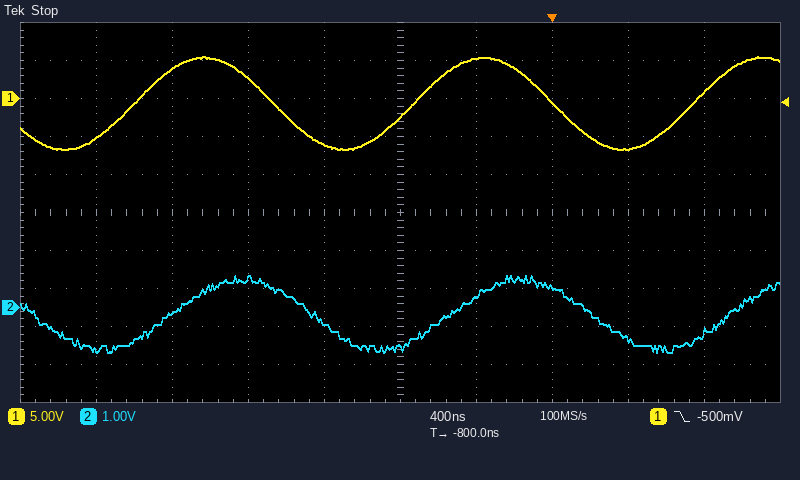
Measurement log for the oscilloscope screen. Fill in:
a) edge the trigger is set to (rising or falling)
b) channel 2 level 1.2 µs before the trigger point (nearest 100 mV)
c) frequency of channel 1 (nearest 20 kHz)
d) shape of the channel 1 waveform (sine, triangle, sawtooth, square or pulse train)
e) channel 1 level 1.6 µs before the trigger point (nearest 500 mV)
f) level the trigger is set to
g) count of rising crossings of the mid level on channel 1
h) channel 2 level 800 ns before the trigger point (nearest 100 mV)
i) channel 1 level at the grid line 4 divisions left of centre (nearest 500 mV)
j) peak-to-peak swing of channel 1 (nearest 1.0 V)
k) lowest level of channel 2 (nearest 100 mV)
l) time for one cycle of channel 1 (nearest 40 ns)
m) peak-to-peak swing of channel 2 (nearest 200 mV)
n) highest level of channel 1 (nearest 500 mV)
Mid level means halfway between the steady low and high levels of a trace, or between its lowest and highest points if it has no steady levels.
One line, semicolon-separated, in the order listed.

falling; -400 mV; 680 kHz; sine; 2.5 V; -500 mV; 3; -1.1 V; -5.0 V; 12.0 V; -1.2 V; 1.48 µs; 2.0 V; 5.5 V
